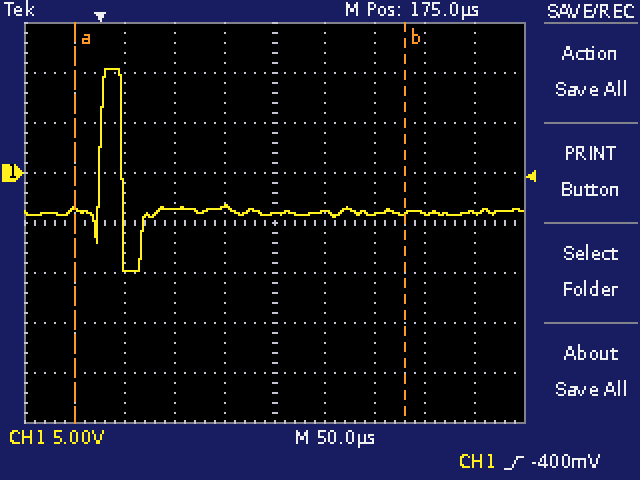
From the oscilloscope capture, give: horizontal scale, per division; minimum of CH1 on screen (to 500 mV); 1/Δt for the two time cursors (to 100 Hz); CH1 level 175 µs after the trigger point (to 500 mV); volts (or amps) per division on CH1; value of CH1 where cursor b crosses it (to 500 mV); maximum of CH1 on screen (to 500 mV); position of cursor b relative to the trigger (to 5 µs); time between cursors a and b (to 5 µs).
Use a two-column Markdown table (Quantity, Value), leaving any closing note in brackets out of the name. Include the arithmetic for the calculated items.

| Quantity | Value |
|---|---|
| horizontal scale, per division | 50 µs |
| minimum of CH1 on screen | -10.0 V |
| 1/Δt for the two time cursors | 1 / 330 µs ≈ 3.0 kHz |
| CH1 level 175 µs after the trigger point | -4.0 V |
| volts (or amps) per division on CH1 | 5 V |
| value of CH1 where cursor b crosses it | -4.0 V |
| maximum of CH1 on screen | 10.5 V |
| position of cursor b relative to the trigger | +305 µs |
| time between cursors a and b | 330 µs |
